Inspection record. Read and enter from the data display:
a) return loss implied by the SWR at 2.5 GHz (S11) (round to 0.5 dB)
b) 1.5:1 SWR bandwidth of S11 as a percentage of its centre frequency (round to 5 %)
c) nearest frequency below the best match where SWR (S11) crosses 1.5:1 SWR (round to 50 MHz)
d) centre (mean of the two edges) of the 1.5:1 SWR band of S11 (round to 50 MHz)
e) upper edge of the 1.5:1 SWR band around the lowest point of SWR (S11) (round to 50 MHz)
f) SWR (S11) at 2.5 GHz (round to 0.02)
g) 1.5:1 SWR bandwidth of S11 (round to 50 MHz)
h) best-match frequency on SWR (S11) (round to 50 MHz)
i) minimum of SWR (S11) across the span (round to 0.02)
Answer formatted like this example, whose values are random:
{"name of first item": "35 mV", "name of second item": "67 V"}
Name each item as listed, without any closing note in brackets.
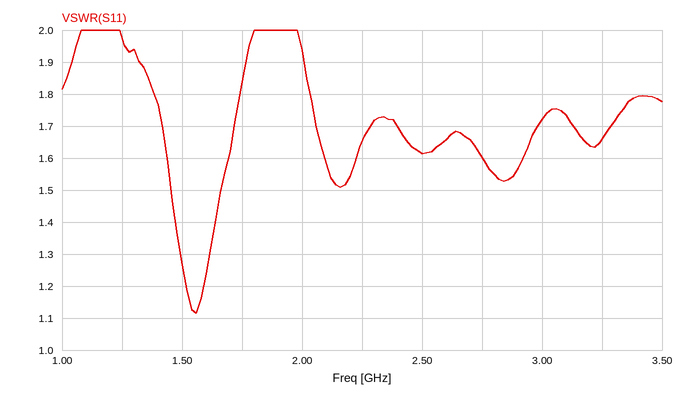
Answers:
{"return loss implied by the SWR at 2.5 GHz (S11)": "12.5 dB", "1.5:1 SWR bandwidth of S11 as a percentage of its centre frequency": "15 %", "nearest frequency below the best match where SWR (S11) crosses 1.5:1 SWR": "1.45 GHz", "centre (mean of the two edges) of the 1.5:1 SWR band of S11": "1.55 GHz", "upper edge of the 1.5:1 SWR band around the lowest point of SWR (S11)": "1.65 GHz", "SWR (S11) at 2.5 GHz": "1.62", "1.5:1 SWR bandwidth of S11": "200 MHz", "best-match frequency on SWR (S11)": "1.55 GHz", "minimum of SWR (S11) across the span": "1.12"}
